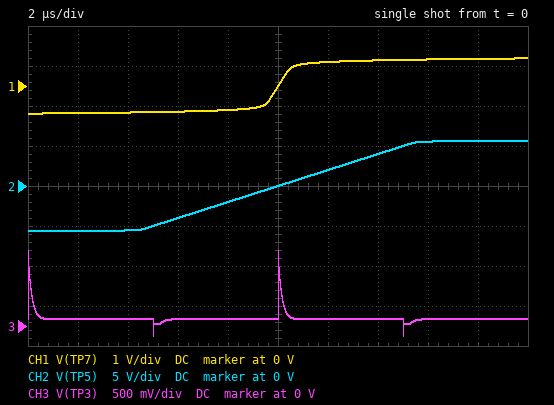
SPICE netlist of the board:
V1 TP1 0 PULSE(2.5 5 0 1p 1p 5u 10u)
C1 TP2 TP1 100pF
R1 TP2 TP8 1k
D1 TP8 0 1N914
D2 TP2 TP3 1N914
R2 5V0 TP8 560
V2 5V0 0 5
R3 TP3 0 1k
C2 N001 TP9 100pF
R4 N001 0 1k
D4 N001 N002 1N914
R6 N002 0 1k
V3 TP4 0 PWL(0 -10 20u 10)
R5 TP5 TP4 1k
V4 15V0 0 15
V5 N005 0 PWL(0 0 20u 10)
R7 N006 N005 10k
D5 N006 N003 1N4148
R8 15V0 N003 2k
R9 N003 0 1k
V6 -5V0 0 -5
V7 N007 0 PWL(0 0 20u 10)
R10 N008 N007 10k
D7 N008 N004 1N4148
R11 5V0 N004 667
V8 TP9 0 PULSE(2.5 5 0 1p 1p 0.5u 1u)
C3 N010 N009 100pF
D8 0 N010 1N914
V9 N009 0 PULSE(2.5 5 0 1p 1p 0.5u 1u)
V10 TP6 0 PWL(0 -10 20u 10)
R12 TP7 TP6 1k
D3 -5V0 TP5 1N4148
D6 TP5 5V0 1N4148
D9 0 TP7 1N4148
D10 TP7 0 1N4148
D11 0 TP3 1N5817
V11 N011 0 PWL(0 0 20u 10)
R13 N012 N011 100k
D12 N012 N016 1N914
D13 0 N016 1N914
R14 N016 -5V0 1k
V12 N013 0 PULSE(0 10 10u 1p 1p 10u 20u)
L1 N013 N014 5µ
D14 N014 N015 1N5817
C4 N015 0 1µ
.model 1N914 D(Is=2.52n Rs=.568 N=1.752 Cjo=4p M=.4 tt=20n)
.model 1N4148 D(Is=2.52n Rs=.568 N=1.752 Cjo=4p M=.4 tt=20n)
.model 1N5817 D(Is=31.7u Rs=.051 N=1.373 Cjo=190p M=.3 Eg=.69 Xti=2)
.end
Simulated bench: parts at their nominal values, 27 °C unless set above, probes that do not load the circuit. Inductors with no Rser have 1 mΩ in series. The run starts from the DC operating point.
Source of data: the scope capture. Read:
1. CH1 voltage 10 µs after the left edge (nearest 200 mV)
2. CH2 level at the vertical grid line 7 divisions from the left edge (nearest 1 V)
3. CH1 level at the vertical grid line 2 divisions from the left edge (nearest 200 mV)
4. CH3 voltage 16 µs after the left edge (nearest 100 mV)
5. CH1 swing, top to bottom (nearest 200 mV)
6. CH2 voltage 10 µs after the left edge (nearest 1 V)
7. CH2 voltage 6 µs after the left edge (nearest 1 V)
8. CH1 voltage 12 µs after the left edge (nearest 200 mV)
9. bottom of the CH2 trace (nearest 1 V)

0 V
4 V
-600 mV
100 mV
1.4 V
0 V
-4 V
600 mV
-6 V
